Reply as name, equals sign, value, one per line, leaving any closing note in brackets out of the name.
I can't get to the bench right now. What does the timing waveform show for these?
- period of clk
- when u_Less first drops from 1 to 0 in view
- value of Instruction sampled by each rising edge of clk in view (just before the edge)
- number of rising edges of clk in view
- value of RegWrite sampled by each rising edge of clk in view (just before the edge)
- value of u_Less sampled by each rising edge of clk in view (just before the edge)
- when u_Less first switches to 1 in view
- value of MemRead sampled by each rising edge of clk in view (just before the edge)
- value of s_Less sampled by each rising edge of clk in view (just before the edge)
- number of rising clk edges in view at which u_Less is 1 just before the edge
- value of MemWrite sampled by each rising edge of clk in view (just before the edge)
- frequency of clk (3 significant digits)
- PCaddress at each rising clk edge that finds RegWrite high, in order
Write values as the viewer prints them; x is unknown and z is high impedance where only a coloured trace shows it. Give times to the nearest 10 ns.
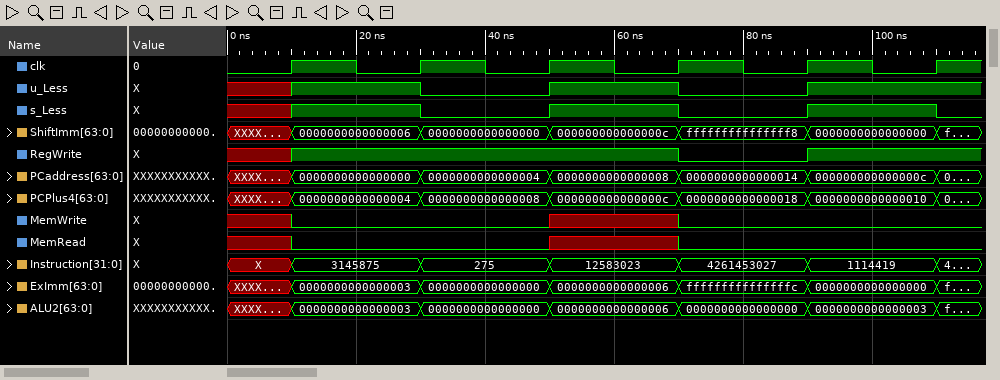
period of clk = 20 ns
when u_Less first drops from 1 to 0 in view = 30 ns
value of Instruction sampled by each rising edge of clk in view = X, 3145875, 275, 12583023, 4261453027, 1114419
number of rising edges of clk in view = 6
value of RegWrite sampled by each rising edge of clk in view = x 1 1 1 0 1
value of u_Less sampled by each rising edge of clk in view = x 1 0 1 0 1
when u_Less first switches to 1 in view = 10 ns
value of MemRead sampled by each rising edge of clk in view = x 0 0 x 0 0
value of s_Less sampled by each rising edge of clk in view = x 1 0 1 0 1
number of rising clk edges in view at which u_Less is 1 just before the edge = 3
value of MemWrite sampled by each rising edge of clk in view = x 0 0 x 0 0
frequency of clk = 50.0 MHz
PCaddress at each rising clk edge that finds RegWrite high, in order = 0000000000000000, 0000000000000004, 0000000000000008, 000000000000000c
